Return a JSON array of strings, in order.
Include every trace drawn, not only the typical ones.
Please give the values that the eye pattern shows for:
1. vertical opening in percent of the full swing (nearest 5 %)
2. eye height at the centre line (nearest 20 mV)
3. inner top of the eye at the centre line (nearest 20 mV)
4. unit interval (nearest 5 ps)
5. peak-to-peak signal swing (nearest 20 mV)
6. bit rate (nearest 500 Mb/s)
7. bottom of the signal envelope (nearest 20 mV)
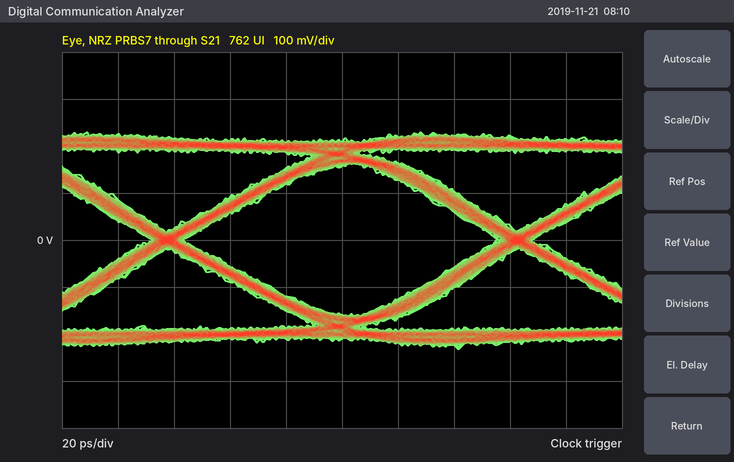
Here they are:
["70 %", "320 mV", "160 mV", "125 ps", "460 mV", "8.0 Gb/s", "-240 mV"]
